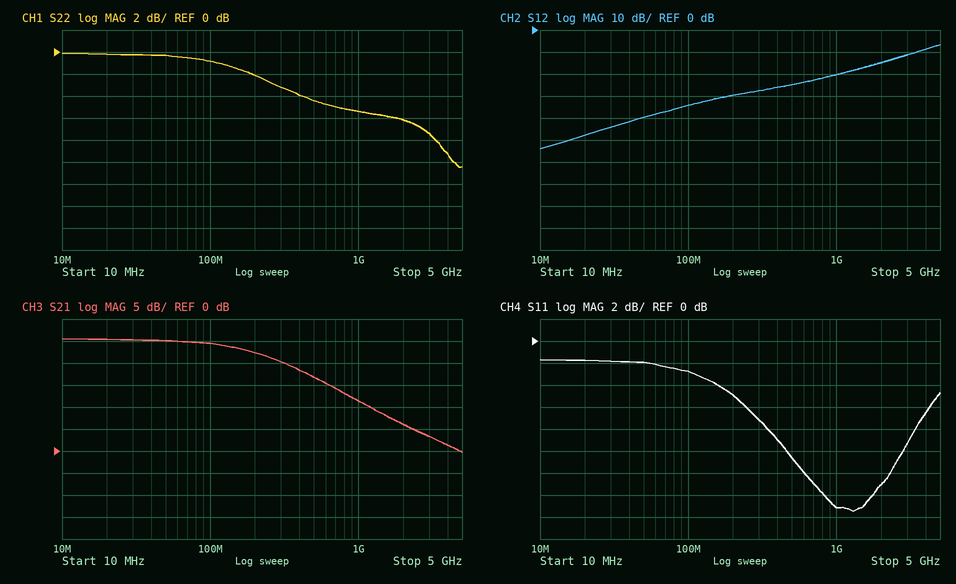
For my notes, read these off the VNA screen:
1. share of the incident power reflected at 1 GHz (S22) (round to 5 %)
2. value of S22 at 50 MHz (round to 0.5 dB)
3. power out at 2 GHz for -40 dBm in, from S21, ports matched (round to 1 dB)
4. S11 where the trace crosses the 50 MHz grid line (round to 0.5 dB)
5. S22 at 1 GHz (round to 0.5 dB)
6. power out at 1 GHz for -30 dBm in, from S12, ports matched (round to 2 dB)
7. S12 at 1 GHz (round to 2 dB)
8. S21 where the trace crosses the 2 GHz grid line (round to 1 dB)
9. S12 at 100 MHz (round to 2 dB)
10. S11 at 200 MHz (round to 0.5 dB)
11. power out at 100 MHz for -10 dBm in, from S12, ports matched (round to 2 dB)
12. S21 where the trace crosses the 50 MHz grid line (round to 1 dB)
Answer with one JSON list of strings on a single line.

["30 %", "-0.5 dB", "-34 dBm", "-2.0 dB", "-5.5 dB", "-50 dBm", "-20 dB", "6 dB", "-34 dB", "-5.0 dB", "-44 dBm", "25 dB"]
